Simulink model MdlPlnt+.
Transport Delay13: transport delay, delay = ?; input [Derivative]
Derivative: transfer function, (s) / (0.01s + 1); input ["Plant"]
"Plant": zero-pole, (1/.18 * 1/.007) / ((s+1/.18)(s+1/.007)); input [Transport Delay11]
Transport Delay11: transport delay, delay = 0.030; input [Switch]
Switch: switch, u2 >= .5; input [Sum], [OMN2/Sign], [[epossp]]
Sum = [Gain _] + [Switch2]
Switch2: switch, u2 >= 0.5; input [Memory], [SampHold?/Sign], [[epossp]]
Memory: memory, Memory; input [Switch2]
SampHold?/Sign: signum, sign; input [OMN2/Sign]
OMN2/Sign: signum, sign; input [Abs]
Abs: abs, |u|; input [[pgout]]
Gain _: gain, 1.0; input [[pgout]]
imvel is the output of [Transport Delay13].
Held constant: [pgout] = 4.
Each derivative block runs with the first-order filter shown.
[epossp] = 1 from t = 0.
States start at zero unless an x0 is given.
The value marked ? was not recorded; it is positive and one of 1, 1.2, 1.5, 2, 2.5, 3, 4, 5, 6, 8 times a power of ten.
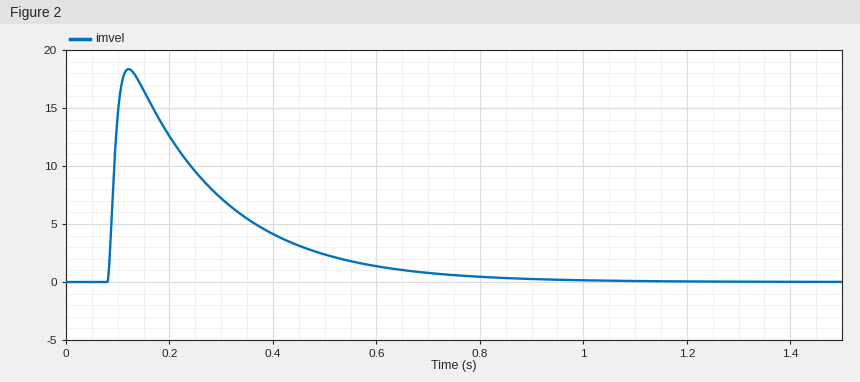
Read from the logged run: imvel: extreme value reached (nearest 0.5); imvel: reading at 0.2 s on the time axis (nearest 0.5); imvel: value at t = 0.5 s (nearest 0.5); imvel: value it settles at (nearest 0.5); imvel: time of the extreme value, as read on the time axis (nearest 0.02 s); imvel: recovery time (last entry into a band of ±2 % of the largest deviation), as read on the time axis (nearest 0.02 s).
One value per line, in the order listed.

18.5
12.5
2.5
0.0
0.12 s
0.84 s
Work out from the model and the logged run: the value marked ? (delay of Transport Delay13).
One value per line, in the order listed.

0.05
